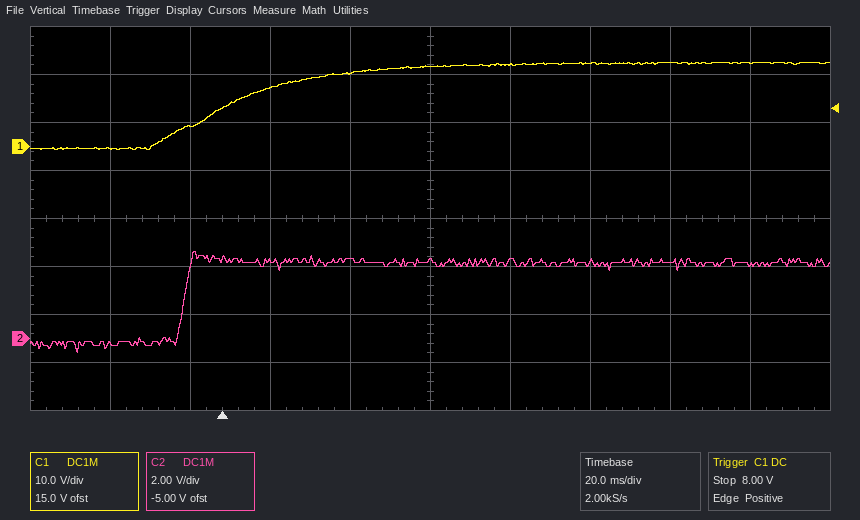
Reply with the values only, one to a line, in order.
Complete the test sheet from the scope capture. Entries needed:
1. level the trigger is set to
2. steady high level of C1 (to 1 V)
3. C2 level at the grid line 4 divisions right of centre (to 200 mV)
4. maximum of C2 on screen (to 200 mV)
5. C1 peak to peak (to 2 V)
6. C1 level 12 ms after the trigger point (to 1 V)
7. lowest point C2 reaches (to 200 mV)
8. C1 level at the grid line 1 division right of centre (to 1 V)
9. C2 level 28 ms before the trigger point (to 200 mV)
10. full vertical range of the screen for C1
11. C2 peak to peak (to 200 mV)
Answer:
8.00 V
17 V
3.0 V
3.6 V
18 V
12 V
-600 mV
17 V
-200 mV
80 V
4.2 V
